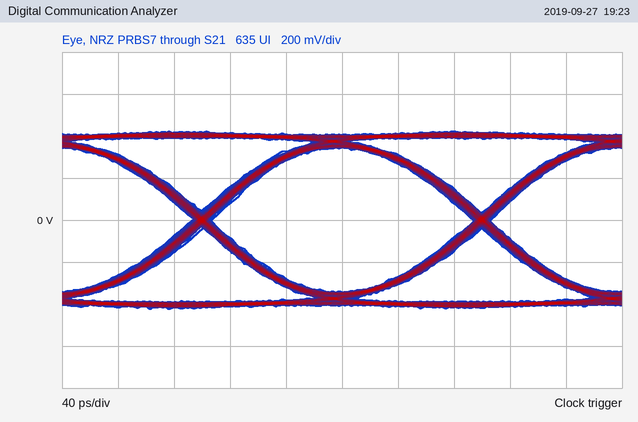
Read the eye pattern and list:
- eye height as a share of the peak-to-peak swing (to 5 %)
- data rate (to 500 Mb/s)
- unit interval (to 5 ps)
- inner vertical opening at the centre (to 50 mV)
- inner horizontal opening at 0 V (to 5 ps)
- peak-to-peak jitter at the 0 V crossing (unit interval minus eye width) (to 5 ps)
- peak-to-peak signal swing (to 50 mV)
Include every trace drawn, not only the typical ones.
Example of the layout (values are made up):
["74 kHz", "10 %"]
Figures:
["80 %", "5.0 Gb/s", "200 ps", "700 mV", "185 ps", "15 ps", "850 mV"]
